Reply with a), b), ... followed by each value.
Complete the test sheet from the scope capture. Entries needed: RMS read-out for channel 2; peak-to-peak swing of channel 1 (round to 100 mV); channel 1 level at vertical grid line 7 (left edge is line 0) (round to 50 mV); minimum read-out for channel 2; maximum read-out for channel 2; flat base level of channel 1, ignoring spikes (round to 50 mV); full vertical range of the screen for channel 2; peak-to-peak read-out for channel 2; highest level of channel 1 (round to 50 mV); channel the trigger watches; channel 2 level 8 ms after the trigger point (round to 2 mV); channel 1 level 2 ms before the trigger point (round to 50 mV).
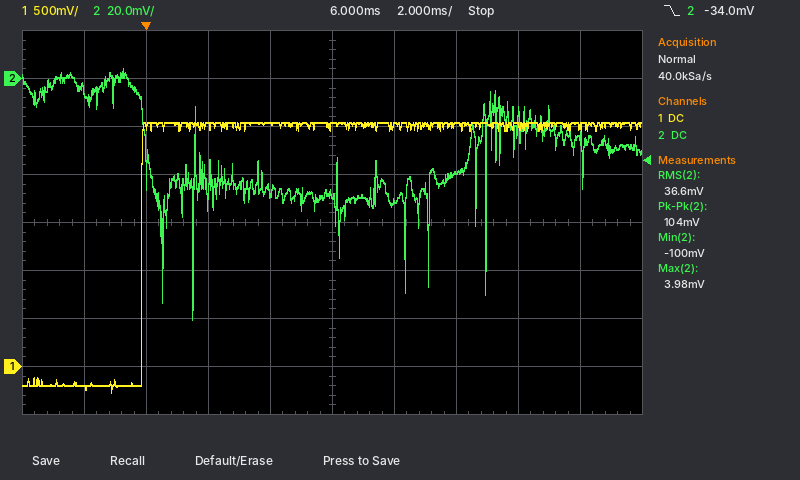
a) 36.6 mV
b) 2.80 V
c) 2.50 V
d) -100 mV
e) 3.98 mV
f) -200 mV
g) 160 mV
h) 104 mV
i) 2.55 V
j) channel 2
k) -52 mV
l) -200 mV
